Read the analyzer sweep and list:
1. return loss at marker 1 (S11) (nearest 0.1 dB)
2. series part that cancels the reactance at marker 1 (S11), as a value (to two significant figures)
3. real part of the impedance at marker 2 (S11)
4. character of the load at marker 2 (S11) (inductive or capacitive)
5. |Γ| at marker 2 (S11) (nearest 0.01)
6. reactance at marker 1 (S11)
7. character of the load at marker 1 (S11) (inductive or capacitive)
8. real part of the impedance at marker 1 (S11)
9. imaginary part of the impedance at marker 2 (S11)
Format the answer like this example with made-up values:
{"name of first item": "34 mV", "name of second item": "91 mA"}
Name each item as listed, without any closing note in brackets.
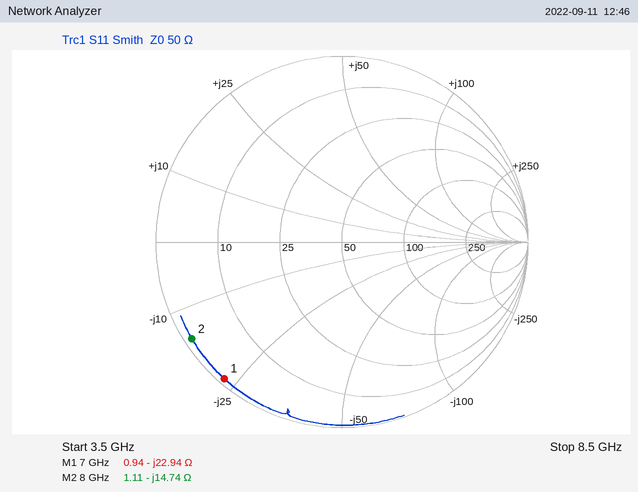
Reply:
{"return loss at marker 1 (S11)": "0.3 dB", "series part that cancels the reactance at marker 1 (S11), as a value": "520 pH", "real part of the impedance at marker 2": "1.11 Ω", "character of the load at marker 2 (S11)": "capacitive", "|Γ| at marker 2 (S11)": "0.96", "reactance at marker 1": "-22.94 Ω", "character of the load at marker 1 (S11)": "capacitive", "real part of the impedance at marker 1": "0.94 Ω", "imaginary part of the impedance at marker 2": "-14.74 Ω"}
